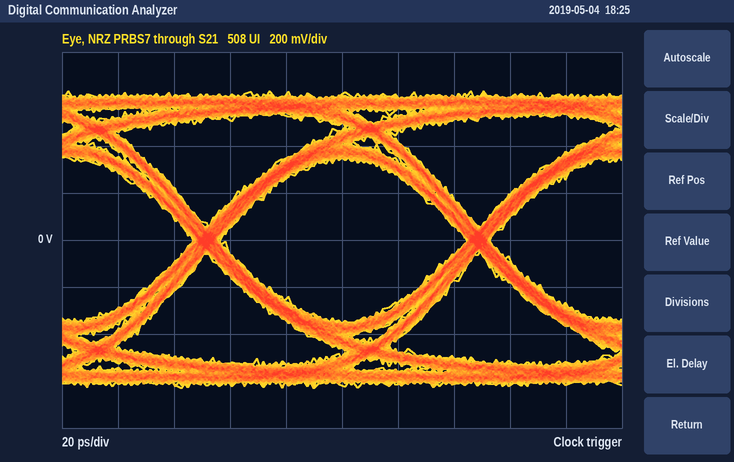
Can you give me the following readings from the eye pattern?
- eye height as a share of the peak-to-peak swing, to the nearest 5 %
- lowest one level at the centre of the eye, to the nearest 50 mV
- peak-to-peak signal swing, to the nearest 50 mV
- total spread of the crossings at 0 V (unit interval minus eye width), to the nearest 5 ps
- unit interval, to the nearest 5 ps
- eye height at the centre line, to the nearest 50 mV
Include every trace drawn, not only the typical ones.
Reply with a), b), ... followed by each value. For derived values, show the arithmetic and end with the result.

a) 700 mV / 1.25 V ≈ 56.0 %, so 55 % to the nearest 5 %
b) 350 mV
c) 1.25 V
d) 10 ps
e) 95 ps
f) 700 mV
